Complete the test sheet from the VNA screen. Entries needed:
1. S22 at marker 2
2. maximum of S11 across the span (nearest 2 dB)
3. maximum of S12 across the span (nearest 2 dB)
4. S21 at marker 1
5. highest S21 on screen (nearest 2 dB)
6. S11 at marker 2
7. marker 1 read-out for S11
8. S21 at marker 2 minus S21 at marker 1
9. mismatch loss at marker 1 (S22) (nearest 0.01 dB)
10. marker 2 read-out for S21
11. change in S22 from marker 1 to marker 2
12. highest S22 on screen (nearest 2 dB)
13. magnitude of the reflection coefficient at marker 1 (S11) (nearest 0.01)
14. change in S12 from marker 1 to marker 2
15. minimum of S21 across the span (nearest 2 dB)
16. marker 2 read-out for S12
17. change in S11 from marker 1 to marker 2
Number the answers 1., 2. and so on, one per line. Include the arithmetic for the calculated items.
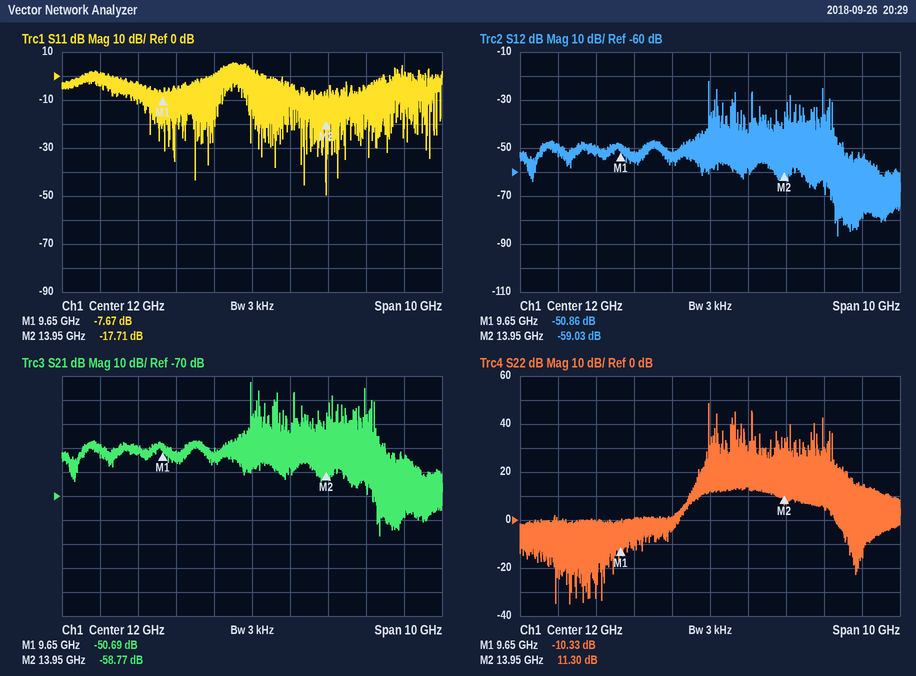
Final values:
1. 11.30 dB
2. 6 dB
3. -22 dB
4. -50.69 dB
5. -22 dB
6. -17.71 dB
7. -7.67 dB
8. -58.77 − (-50.69) = -8.08 dB
9. −10 log10(1 − 10^(-10.33/10)) ≈ 0.42 dB
10. -58.77 dB
11. 11.3 − (-10.33) = 21.63 dB
12. 48 dB
13. 10^(-7.67/20) ≈ 0.41
14. -59.03 − (-50.86) = -8.17 dB
15. -86 dB
16. -59.03 dB
17. -17.71 − (-7.67) = -10.04 dB
